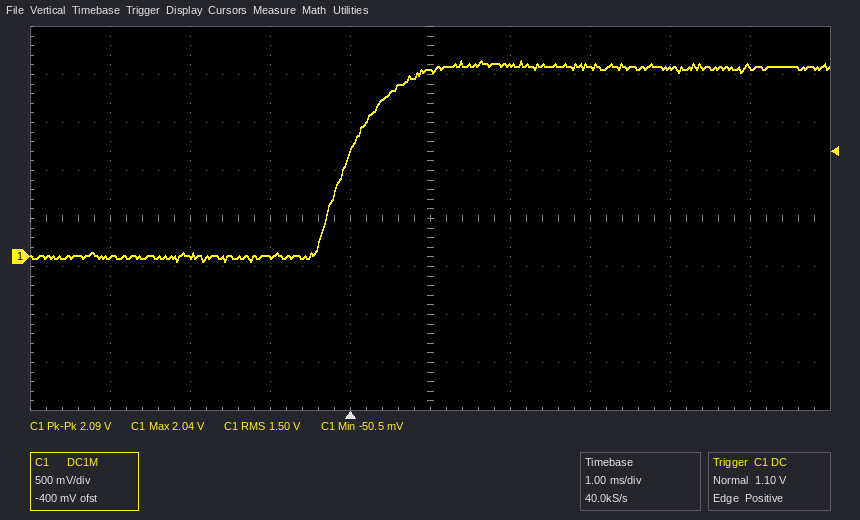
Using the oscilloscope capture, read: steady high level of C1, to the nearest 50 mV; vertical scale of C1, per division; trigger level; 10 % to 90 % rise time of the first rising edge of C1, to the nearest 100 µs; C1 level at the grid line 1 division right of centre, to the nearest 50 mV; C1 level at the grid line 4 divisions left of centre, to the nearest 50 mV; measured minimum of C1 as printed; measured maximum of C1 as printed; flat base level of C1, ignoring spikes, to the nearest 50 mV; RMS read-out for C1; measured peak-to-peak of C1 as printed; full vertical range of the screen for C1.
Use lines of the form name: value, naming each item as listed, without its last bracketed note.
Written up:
steady high level of C1, to the nearest 50 mV: 2.00 V
vertical scale of C1, per division: 500 mV
trigger level: 1.10 V
10 % to 90 % rise time of the first rising edge of C1, to the nearest 100 µs: 1.0 ms
C1 level at the grid line 1 division right of centre, to the nearest 50 mV: 2.00 V
C1 level at the grid line 4 divisions left of centre, to the nearest 50 mV: 0 mV
measured minimum of C1 as printed: -50.5 mV
measured maximum of C1 as printed: 2.04 V
flat base level of C1, ignoring spikes, to the nearest 50 mV: 0 mV
RMS read-out for C1: 1.50 V
measured peak-to-peak of C1 as printed: 2.09 V
full vertical range of the screen for C1: 4 V
